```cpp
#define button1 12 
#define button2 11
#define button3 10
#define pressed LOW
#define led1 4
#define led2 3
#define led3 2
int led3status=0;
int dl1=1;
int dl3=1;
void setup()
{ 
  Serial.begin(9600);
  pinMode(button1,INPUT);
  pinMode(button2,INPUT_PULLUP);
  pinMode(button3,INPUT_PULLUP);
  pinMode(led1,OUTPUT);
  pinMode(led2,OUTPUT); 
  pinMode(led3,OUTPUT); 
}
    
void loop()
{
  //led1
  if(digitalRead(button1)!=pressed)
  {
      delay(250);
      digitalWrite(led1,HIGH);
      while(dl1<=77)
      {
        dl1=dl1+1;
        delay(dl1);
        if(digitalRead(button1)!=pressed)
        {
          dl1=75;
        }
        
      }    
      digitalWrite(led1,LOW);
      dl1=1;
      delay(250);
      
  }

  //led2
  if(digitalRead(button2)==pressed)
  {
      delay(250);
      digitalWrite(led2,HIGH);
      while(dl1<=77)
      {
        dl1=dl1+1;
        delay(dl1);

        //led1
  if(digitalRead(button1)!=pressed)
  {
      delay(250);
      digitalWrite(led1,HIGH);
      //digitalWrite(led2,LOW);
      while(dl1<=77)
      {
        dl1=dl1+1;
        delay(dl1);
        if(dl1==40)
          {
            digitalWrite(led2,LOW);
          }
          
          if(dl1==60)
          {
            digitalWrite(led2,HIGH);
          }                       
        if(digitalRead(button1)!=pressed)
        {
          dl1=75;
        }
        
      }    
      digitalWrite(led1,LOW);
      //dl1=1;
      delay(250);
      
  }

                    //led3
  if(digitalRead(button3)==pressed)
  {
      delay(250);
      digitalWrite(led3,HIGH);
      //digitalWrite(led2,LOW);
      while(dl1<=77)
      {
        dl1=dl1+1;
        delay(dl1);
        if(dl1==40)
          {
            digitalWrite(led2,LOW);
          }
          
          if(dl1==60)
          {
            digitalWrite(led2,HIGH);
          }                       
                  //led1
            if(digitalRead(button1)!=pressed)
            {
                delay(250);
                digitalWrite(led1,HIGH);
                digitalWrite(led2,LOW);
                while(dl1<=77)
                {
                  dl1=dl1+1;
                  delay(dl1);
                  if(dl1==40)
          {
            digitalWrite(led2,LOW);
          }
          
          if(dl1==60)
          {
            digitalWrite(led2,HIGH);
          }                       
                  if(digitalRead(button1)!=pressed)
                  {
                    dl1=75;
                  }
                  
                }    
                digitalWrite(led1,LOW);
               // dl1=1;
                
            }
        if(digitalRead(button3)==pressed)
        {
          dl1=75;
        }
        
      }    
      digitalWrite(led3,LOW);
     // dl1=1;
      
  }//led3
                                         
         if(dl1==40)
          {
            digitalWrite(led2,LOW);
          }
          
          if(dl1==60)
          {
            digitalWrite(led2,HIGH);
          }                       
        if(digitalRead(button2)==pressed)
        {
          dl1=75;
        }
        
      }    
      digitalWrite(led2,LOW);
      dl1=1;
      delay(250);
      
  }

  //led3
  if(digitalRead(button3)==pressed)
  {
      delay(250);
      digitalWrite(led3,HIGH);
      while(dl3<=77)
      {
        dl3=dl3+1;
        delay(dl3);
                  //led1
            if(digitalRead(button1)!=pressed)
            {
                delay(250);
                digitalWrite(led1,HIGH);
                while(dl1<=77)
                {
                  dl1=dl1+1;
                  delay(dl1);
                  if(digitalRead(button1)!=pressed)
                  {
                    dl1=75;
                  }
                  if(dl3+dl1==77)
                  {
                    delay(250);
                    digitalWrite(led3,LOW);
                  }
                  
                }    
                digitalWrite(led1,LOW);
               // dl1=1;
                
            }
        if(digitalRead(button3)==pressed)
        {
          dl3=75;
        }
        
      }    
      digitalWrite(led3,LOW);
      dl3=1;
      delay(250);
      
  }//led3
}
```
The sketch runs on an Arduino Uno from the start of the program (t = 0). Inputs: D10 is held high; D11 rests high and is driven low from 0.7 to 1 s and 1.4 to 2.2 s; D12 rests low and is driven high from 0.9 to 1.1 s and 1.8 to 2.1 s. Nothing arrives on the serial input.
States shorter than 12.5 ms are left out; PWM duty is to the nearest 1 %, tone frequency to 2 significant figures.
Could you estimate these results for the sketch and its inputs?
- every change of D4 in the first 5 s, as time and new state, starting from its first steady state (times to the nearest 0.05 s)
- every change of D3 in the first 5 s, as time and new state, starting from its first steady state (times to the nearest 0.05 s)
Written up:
0 s low; 1.2 s high; 2.3 s low
0 s low; 0.95 s high; 2.55 s low
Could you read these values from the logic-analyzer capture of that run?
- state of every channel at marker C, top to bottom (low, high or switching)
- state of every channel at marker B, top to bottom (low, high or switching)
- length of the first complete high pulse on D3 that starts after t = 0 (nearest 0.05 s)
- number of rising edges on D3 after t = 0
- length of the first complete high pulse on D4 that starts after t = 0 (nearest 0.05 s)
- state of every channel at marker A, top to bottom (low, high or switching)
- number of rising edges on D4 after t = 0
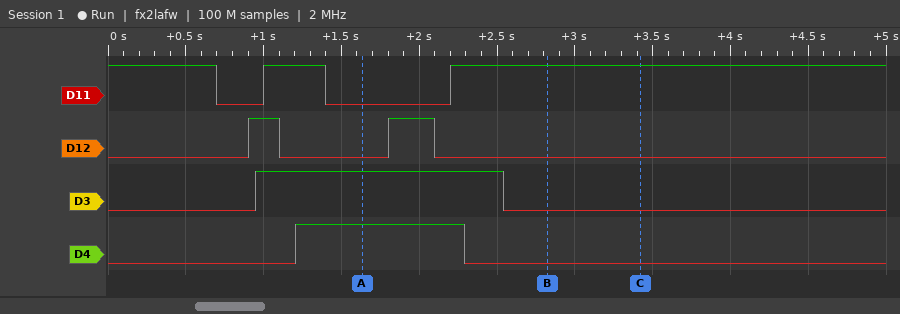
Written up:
D11 high, D12 low, D3 low, D4 low
D11 high, D12 low, D3 low, D4 low
1.60 s
1
1.10 s
D11 low, D12 low, D3 high, D4 high
1
